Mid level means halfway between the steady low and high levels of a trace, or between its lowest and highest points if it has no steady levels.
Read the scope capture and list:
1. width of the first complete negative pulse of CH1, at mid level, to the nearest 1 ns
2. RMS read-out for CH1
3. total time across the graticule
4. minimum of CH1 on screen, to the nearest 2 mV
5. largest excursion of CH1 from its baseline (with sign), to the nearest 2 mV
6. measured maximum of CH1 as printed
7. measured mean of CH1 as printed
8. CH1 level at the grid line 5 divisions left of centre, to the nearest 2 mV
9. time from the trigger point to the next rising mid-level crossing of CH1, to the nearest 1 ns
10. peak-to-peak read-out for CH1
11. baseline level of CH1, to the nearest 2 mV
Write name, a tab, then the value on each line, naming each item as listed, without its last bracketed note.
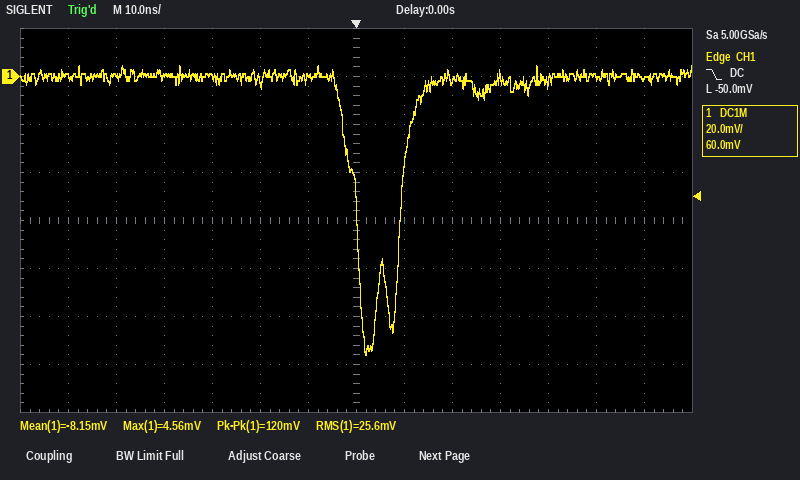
width of the first complete negative pulse of CH1, at mid level, to the nearest 1 ns	9 ns
RMS read-out for CH1	25.6 mV
total time across the graticule	140 ns
minimum of CH1 on screen, to the nearest 2 mV	-116 mV
largest excursion of CH1 from its baseline (with sign), to the nearest 2 mV	-116 mV
measured maximum of CH1 as printed	4.56 mV
measured mean of CH1 as printed	-8.15 mV
CH1 level at the grid line 5 divisions left of centre, to the nearest 2 mV	0 mV
time from the trigger point to the next rising mid-level crossing of CH1, to the nearest 1 ns	9 ns
peak-to-peak read-out for CH1	120 mV
baseline level of CH1, to the nearest 2 mV	0 mV
